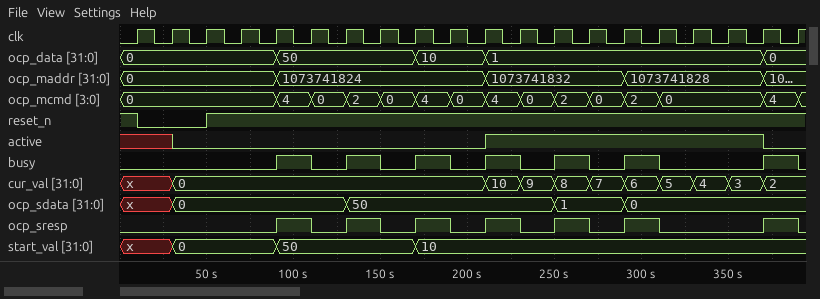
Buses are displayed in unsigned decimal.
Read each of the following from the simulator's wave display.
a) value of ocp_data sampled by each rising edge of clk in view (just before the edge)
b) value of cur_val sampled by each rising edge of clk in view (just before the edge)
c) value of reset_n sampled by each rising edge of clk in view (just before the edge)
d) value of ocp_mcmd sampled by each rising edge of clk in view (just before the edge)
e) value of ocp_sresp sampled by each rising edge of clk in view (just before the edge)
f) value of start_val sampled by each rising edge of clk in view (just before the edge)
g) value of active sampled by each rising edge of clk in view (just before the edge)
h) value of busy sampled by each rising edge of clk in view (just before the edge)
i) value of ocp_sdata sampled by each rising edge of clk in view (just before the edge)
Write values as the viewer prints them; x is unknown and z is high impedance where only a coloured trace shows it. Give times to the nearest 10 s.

0, 0, 0, 0, 0, 50, 50, 50, 50, 10, 10, 1, 1, 1, 1, 1, 1, 1, 1, 0
x, x, 0, 0, 0, 0, 0, 0, 0, 0, 0, 10, 9, 8, 7, 6, 5, 4, 3, 2
1 0 0 1 1 1 1 1 1 1 1 1 1 1 1 1 1 1 1 1
0, 0, 0, 0, 0, 4, 0, 2, 0, 4, 0, 4, 0, 2, 0, 2, 0, 0, 0, 4
0 0 0 0 0 1 0 1 0 1 0 1 0 1 0 1 0 0 0 1
x, x, 0, 0, 0, 50, 50, 50, 50, 10, 10, 10, 10, 10, 10, 10, 10, 10, 10, 10
x x 0 0 0 0 0 0 0 0 0 1 1 1 1 1 1 1 1 0
0 0 0 0 0 1 0 1 0 1 0 1 0 1 0 1 0 0 0 1
x, x, 0, 0, 0, 0, 0, 50, 50, 50, 50, 50, 50, 1, 1, 0, 0, 0, 0, 0
